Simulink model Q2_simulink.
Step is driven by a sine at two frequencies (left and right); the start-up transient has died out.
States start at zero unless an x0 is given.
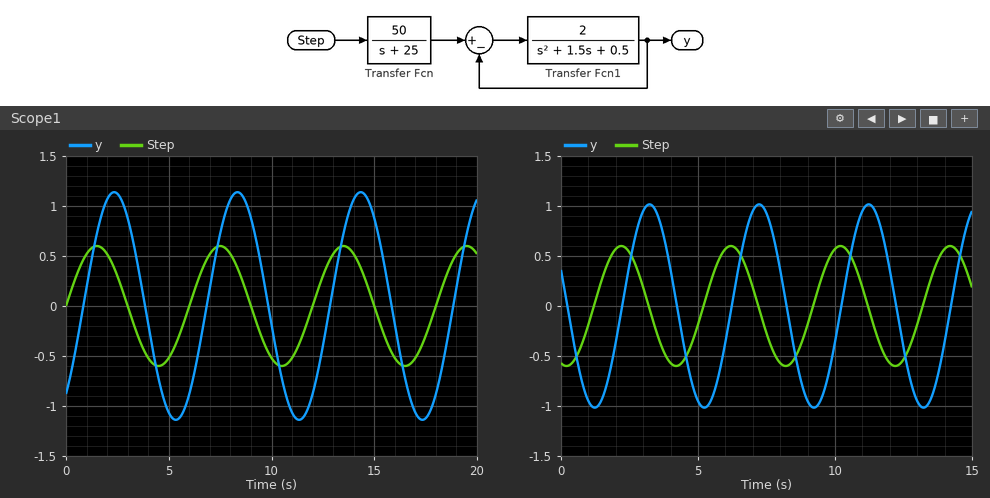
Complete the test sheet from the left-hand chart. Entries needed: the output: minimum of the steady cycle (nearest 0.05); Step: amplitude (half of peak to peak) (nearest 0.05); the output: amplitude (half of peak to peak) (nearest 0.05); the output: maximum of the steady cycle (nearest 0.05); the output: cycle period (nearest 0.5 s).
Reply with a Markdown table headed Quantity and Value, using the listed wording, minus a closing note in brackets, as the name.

| Quantity | Value |
|---|---|
| the output: minimum of the steady cycle | -1.15 |
| Step: amplitude (half of peak to peak) | 0.60 |
| the output: amplitude (half of peak to peak) | 1.15 |
| the output: maximum of the steady cycle | 1.15 |
| the output: cycle period | 6.0 s |
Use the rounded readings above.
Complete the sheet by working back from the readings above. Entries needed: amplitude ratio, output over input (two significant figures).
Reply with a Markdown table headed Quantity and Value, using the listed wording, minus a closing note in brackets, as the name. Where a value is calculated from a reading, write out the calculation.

| Quantity | Value |
|---|---|
| amplitude ratio, output over input | 1.15 / 0.6 = 1.9 |
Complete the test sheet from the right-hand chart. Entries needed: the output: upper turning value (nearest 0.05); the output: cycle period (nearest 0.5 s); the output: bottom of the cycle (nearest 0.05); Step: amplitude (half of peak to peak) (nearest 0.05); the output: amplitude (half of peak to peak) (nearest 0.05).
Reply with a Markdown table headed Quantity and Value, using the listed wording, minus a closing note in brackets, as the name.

| Quantity | Value |
|---|---|
| the output: upper turning value | 1.00 |
| the output: cycle period | 4.0 s |
| the output: bottom of the cycle | -1.00 |
| Step: amplitude (half of peak to peak) | 0.60 |
| the output: amplitude (half of peak to peak) | 1.00 |
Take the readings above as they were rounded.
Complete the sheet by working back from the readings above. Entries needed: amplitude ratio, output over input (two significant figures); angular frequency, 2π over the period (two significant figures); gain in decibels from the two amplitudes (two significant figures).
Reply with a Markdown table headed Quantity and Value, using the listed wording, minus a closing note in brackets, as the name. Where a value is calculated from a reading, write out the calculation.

| Quantity | Value |
|---|---|
| amplitude ratio, output over input | 1 / 0.6 = 1.7 |
| angular frequency, 2π over the period | 2π / 4 = 1.6 rad/s |
| gain in decibels from the two amplitudes | 20 log10(1 / 0.6) = 4.4 dB |
